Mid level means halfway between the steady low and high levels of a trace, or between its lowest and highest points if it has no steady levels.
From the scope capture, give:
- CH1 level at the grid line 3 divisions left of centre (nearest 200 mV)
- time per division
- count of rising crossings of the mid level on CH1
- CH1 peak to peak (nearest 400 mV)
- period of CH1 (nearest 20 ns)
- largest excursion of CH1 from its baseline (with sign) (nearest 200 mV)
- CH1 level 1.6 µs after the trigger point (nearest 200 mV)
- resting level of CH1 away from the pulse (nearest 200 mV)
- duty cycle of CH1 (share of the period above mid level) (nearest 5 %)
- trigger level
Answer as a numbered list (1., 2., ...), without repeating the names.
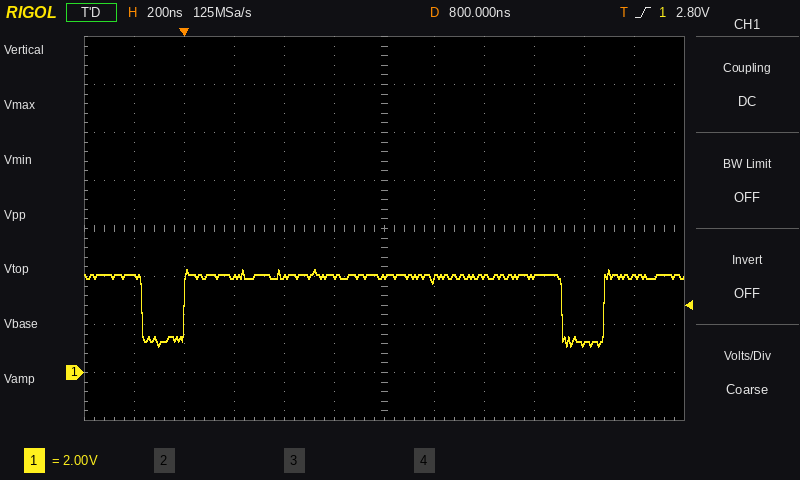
1. 4.0 V
2. 200 ns
3. 2
4. 3.2 V
5. 1.68 µs
6. -3.0 V
7. 1.2 V
8. 4.0 V
9. 90 %
10. 2.80 V
